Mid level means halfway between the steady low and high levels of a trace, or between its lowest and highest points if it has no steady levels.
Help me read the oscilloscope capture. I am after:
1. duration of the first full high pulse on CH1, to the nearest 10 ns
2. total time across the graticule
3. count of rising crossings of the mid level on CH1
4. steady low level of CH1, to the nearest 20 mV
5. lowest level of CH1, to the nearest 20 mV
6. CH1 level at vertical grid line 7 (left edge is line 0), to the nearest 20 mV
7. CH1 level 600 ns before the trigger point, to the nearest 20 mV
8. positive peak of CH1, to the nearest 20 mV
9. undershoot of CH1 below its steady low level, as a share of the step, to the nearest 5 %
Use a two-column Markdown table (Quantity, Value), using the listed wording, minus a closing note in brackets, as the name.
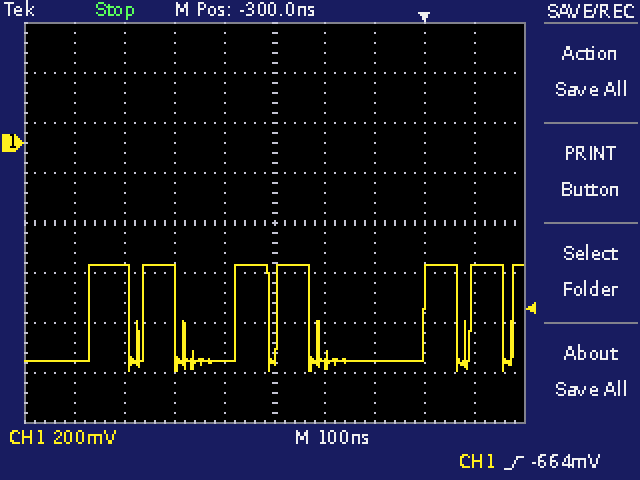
| Quantity | Value |
|---|---|
| duration of the first full high pulse on CH1, to the nearest 10 ns | 80 ns |
| total time across the graticule | 1 µs |
| count of rising crossings of the mid level on CH1 | 7 |
| steady low level of CH1, to the nearest 20 mV | -880 mV |
| lowest level of CH1, to the nearest 20 mV | -920 mV |
| CH1 level at vertical grid line 7 (left edge is line 0), to the nearest 20 mV | -880 mV |
| CH1 level 600 ns before the trigger point, to the nearest 20 mV | -480 mV |
| positive peak of CH1, to the nearest 20 mV | -480 mV |
| undershoot of CH1 below its steady low level, as a share of the step, to the nearest 5 % | 10 % |
